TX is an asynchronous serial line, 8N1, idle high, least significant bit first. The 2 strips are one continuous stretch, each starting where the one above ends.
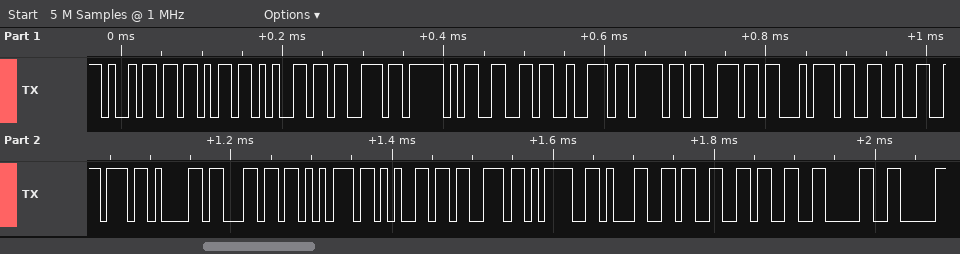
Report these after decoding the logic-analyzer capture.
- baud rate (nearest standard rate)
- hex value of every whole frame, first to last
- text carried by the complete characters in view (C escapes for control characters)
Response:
115200 baud
69 6B 65 73 5F 66 72 6F 6E 74 26 76 61 6C 75 65 73 3D 31 33 33 30
"ikes_front&values=1330"
